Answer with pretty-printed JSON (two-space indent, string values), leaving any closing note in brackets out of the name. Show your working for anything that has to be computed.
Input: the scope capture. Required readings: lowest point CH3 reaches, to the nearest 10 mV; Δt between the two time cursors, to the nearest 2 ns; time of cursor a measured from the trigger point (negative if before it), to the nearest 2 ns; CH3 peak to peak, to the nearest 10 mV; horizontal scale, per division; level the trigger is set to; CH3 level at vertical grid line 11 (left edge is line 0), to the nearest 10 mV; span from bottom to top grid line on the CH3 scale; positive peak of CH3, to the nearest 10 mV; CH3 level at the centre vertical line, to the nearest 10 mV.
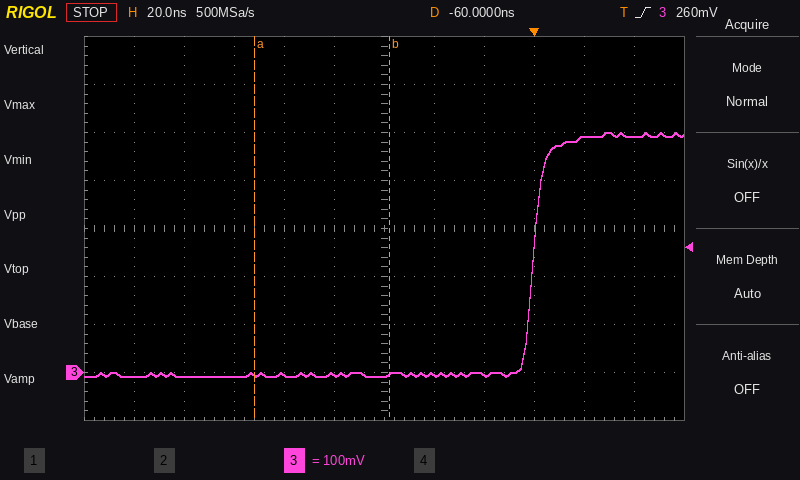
{
  "lowest point CH3 reaches, to the nearest 10 mV": "-10 mV",
  "Δt between the two time cursors, to the nearest 2 ns": "54 ns",
  "time of cursor a measured from the trigger point (negative if before it), to the nearest 2 ns": "-112 ns",
  "CH3 peak to peak, to the nearest 10 mV": "500 mV − (-10 mV) = 510 mV",
  "horizontal scale, per division": "20 ns",
  "level the trigger is set to": "260 mV",
  "CH3 level at vertical grid line 11 (left edge is line 0), to the nearest 10 mV": "490 mV",
  "span from bottom to top grid line on the CH3 scale": "800 mV",
  "positive peak of CH3, to the nearest 10 mV": "500 mV",
  "CH3 level at the centre vertical line, to the nearest 10 mV": "-10 mV"
}
